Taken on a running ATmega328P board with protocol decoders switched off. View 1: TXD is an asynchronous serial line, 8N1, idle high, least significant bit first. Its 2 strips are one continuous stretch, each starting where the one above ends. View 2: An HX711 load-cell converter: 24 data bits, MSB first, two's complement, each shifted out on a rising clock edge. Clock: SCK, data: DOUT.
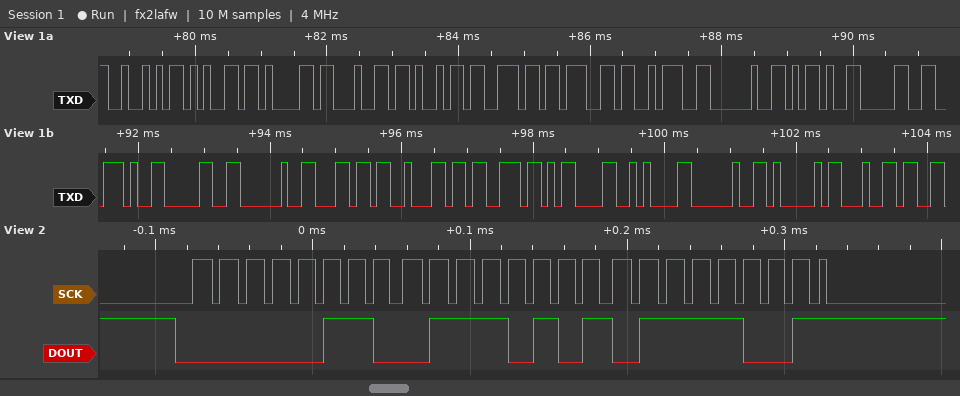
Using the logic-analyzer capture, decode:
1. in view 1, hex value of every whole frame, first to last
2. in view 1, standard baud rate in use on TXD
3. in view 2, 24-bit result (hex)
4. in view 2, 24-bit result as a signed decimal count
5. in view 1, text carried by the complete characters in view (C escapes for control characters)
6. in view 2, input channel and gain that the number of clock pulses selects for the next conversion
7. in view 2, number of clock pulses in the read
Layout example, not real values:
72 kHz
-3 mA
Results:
0x52 0x65 0x61 0x64 0x69 0x6E 0x67 0x3A 0x20 0x2D 0x30 0x2E 0x30 0x20 0x6C 0x62 0x73 0x0D 0x0A 0x20 0x41 0x64
9600 baud
0x067579
423289
"Reading: -0.0 lbs\r\n Ad"
channel A, gain 128
25
